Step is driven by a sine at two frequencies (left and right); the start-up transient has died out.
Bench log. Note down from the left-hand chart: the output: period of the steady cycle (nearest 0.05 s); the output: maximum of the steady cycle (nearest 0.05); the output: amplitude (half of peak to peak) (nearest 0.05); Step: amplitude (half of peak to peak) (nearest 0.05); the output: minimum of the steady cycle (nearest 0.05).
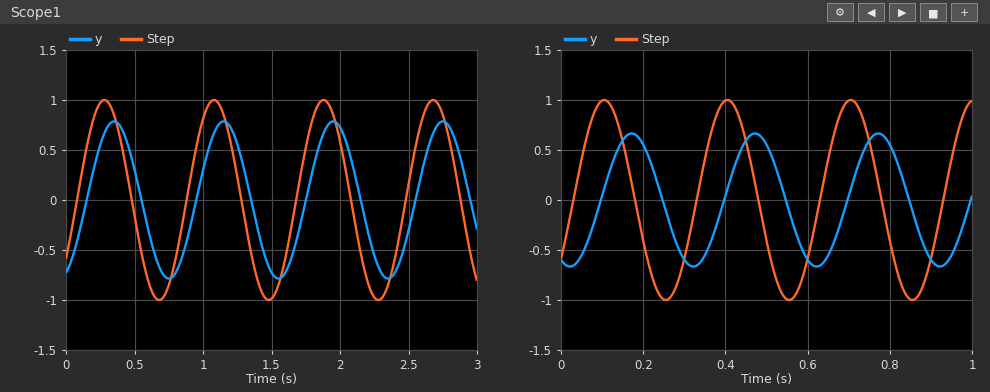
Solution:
0.80 s
0.80
0.80
1.00
-0.80
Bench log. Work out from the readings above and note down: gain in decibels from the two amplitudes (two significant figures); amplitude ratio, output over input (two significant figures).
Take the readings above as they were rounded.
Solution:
-1.9 dB
0.80
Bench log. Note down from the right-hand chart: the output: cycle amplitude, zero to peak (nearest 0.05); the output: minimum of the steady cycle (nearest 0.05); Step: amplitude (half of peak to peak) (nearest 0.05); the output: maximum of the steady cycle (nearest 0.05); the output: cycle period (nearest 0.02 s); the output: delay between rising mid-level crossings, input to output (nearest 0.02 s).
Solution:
0.65
-0.65
1.00
0.65
0.30 s
0.06 s
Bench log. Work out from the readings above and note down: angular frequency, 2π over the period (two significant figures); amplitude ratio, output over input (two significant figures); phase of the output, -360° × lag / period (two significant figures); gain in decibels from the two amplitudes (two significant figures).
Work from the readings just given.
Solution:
21 rad/s
0.65
-72°
-3.7 dB
